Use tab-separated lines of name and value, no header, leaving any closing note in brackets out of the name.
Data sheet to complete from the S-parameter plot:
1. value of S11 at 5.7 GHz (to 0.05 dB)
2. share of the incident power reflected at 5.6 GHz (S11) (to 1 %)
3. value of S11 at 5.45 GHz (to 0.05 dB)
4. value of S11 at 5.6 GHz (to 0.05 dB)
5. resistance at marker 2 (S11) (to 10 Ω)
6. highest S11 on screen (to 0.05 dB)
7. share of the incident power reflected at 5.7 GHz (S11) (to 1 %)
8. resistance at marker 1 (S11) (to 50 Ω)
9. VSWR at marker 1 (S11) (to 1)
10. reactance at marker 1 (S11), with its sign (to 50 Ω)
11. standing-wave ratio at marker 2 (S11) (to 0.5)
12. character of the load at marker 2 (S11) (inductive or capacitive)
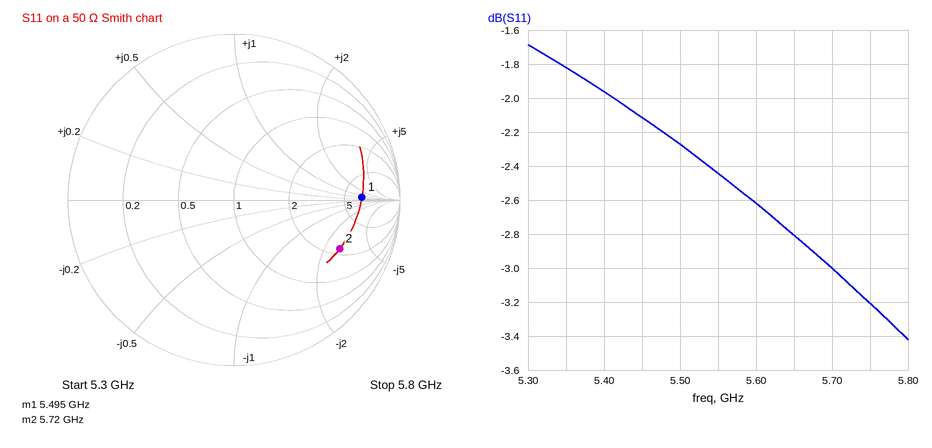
value of S11 at 5.7 GHz	-3.00 dB
share of the incident power reflected at 5.6 GHz (S11)	55 %
value of S11 at 5.45 GHz	-2.10 dB
value of S11 at 5.6 GHz	-2.60 dB
resistance at marker 2 (S11)	120 Ω
highest S11 on screen	-1.70 dB
share of the incident power reflected at 5.7 GHz (S11)	50 %
resistance at marker 1 (S11)	400 Ω
VSWR at marker 1 (S11)	8
reactance at marker 1 (S11), with its sign	+50 Ω
standing-wave ratio at marker 2 (S11)	5.5
character of the load at marker 2 (S11)	capacitive
